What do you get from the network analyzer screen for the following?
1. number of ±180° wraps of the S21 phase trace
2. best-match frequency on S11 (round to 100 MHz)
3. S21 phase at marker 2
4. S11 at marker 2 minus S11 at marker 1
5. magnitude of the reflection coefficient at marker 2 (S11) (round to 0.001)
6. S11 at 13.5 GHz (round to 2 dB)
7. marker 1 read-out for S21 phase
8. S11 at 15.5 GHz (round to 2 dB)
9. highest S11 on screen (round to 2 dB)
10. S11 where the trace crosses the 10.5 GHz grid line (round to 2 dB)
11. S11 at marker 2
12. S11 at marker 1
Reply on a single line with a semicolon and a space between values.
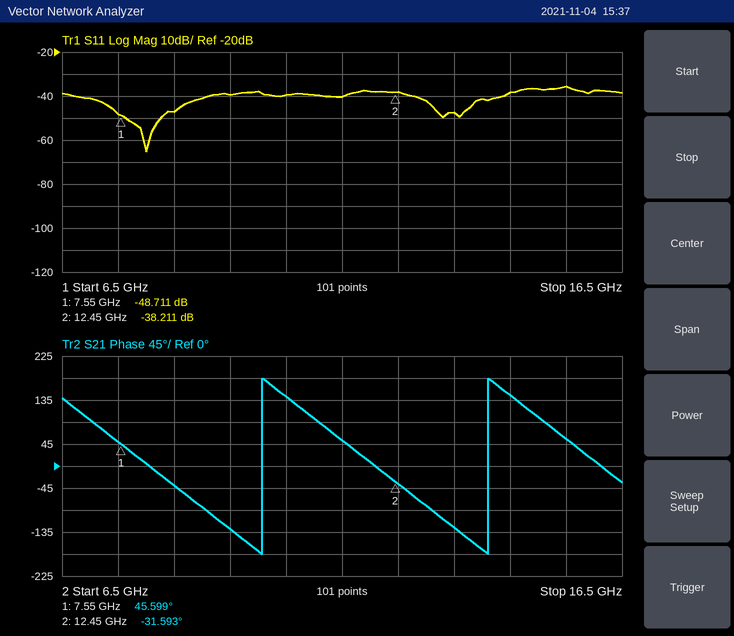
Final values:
2; 8.0 GHz; -31.593°; 10.500 dB; 0.012; -48 dB; 45.599°; -36 dB; -36 dB; -40 dB; -38.211 dB; -48.711 dB
